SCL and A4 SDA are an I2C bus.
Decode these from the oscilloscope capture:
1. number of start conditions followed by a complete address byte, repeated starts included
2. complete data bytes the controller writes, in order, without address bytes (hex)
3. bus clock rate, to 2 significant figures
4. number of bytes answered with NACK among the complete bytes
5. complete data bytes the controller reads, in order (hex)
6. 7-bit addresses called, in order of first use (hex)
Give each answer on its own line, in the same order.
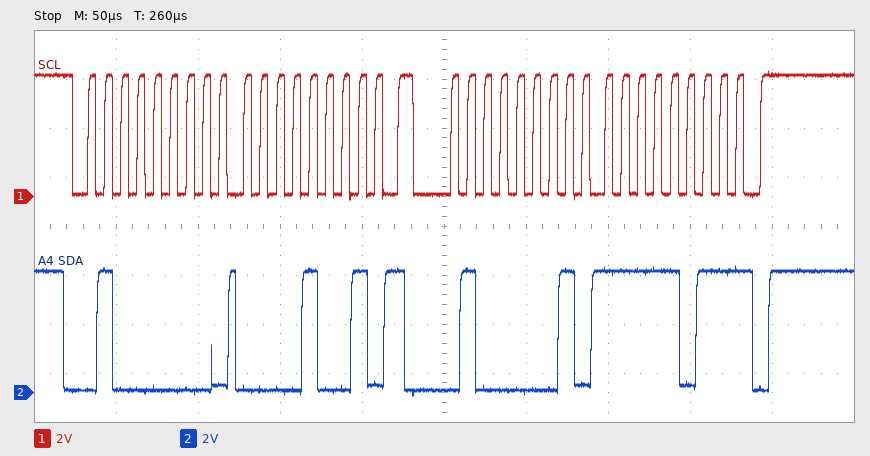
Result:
2
09
100 kHz
1
FB
0x20
